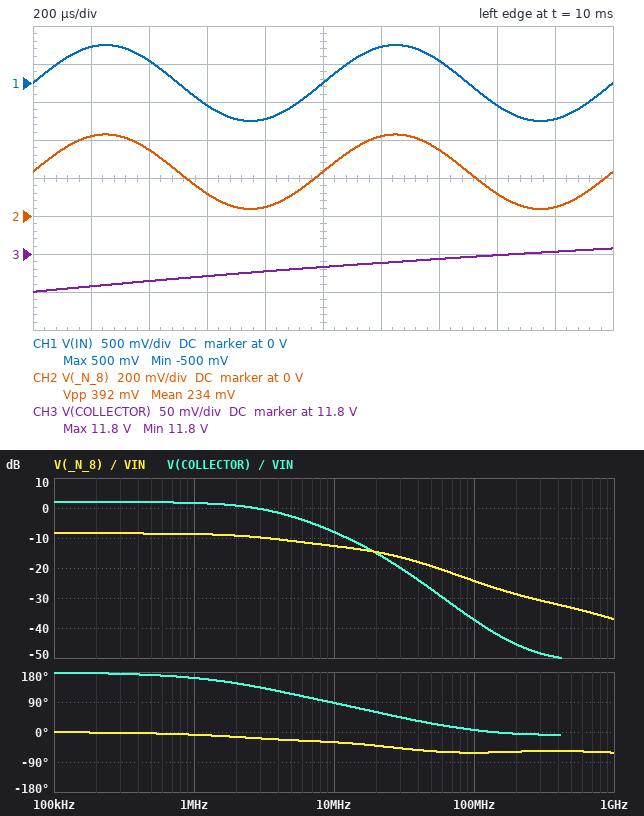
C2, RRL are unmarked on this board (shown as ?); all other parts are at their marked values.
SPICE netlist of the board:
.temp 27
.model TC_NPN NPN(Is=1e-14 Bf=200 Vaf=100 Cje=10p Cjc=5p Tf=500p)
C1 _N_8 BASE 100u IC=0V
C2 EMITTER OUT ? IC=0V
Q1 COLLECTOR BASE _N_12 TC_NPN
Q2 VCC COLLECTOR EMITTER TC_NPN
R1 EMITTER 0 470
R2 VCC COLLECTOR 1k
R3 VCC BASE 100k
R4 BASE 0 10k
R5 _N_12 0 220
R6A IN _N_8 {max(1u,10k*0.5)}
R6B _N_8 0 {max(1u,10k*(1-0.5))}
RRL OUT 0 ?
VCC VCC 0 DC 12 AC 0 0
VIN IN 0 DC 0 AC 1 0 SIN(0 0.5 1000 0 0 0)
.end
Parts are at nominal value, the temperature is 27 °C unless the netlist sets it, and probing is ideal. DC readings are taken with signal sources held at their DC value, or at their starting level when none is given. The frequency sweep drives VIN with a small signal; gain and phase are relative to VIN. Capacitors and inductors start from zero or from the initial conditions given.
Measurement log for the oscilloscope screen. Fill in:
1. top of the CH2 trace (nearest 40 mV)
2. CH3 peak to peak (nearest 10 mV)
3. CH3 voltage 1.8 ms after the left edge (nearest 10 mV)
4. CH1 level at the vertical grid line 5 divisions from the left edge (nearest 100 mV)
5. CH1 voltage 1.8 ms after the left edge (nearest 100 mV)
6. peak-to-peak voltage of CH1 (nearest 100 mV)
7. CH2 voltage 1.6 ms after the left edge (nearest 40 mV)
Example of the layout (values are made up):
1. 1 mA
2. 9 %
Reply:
1. 440 mV
2. 60 mV
3. 11.80 V
4. 0 V
5. -500 mV
6. 1.0 V
7. 120 mV
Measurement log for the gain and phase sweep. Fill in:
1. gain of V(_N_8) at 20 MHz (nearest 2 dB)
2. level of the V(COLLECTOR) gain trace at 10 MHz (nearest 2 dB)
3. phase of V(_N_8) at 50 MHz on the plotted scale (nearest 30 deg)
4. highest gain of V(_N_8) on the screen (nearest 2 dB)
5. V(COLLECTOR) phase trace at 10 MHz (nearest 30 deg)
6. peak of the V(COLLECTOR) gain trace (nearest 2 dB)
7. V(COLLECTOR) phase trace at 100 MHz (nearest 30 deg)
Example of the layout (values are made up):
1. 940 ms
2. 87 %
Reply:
1. -14 dB
2. -8 dB
3. -60 deg
4. -8 dB
5. 90 deg
6. 2 dB
7. 0 deg
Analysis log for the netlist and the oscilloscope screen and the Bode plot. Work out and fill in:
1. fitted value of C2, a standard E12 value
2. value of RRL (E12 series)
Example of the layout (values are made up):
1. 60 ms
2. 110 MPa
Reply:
1. 150 µF
2. 18 Ω
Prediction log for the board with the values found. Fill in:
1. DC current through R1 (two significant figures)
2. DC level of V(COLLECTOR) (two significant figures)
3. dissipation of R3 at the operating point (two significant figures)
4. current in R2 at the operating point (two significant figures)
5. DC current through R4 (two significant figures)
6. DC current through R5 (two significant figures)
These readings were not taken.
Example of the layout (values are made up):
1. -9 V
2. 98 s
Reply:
1. 20 mA
2. 10 V
3. 1.2 mW
4. 1.7 mA
5. 100 µA
6. 1.6 mA
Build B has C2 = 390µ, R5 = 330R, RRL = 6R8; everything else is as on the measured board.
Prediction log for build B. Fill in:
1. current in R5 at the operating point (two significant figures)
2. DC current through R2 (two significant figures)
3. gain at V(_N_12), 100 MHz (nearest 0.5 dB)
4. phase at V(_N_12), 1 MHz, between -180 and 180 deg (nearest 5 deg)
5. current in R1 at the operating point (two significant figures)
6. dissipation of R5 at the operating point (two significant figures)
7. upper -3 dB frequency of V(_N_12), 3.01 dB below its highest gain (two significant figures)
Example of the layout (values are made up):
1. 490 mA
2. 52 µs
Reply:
1. 1.2 mA
2. 1.3 mA
3. -23.0 dB
4. -5 deg
5. 21 mA
6. 450 µW
7. 14 MHz
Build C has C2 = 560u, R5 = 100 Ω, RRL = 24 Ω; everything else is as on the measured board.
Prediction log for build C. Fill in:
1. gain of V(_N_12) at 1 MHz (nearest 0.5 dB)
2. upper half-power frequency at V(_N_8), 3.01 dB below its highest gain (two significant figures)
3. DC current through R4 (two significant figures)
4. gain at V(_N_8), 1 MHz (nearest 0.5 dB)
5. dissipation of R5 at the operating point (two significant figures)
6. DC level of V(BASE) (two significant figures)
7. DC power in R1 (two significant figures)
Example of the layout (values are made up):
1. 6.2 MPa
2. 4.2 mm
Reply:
1. -10.0 dB
2. 2.9 MHz
3. 97 µA
4. -9.5 dB
5. 840 µW
6. 970 mV
7. 150 mW
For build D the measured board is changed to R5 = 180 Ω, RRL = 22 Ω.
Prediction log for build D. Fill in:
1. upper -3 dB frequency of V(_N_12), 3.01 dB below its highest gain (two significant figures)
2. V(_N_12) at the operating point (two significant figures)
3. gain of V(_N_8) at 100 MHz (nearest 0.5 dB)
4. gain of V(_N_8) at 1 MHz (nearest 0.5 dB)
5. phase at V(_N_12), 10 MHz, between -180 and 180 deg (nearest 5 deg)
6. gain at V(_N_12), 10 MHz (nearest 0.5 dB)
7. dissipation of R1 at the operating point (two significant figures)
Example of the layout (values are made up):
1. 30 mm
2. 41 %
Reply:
1. 4.8 MHz
2. 340 mV
3. -25.0 dB
4. -9.0 dB
5. -35 deg
6. -14.5 dB
7. 180 mW
